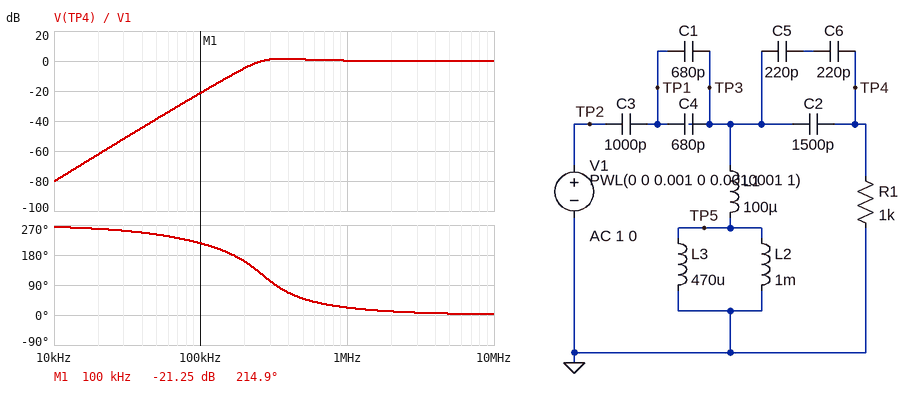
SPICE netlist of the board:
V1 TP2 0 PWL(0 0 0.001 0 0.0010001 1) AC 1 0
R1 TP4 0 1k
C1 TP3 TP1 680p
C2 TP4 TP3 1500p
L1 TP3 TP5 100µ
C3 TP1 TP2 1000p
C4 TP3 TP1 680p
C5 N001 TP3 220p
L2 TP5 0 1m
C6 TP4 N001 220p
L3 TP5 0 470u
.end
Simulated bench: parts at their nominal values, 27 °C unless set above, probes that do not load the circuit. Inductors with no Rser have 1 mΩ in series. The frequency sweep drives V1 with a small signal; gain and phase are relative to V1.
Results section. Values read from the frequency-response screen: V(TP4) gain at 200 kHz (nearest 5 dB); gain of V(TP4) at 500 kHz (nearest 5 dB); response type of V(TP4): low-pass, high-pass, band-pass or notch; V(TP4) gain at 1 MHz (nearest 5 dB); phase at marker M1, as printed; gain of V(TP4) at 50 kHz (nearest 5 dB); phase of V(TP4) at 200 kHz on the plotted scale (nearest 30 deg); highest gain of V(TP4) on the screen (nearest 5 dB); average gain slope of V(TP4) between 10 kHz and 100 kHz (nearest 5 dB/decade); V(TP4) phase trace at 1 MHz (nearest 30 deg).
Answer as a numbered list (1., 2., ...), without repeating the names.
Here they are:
1. -5 dB
2. 0 dB
3. high-pass
4. 0 dB
5. 214.9 deg
6. -40 dB
7. 150 deg
8. 0 dB
9. 60 dB/decade
10. 30 deg
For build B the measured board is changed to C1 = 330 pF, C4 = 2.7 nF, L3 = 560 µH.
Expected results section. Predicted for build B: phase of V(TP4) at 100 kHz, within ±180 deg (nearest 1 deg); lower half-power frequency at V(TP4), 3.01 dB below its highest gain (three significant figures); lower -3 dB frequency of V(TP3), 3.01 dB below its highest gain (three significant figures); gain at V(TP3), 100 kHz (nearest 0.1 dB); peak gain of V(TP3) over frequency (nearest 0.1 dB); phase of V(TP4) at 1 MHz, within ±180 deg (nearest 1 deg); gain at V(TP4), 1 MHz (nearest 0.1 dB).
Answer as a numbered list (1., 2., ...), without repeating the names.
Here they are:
1. -147 deg
2. 196 kHz
3. 191 kHz
4. -14.6 dB
5. 2.7 dB
6. 18 deg
7. 0.2 dB
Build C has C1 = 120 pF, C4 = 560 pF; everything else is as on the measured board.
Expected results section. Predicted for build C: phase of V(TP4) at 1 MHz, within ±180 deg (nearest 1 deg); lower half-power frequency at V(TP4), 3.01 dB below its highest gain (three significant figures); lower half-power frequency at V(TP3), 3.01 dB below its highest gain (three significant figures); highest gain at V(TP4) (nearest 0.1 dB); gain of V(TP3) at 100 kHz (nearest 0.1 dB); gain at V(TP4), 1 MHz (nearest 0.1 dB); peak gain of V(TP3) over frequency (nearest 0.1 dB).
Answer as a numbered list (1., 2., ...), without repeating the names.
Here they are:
1. 29 deg
2. 289 kHz
3. 281 kHz
4. 0.4 dB
5. -21.7 dB
6. 0.2 dB
7. 0.6 dB
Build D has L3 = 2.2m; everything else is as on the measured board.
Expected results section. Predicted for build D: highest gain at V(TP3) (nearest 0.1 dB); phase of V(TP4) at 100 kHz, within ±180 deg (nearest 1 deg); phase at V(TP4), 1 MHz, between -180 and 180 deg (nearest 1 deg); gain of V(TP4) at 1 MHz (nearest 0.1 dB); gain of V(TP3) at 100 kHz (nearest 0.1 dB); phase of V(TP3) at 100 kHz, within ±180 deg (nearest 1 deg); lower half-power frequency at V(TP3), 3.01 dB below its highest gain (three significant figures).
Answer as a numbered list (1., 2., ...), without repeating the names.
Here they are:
1. 0 dB
2. -159 deg
3. 21 deg
4. -0.1 dB
5. -10.9 dB
6. 156 deg
7. 151 kHz
